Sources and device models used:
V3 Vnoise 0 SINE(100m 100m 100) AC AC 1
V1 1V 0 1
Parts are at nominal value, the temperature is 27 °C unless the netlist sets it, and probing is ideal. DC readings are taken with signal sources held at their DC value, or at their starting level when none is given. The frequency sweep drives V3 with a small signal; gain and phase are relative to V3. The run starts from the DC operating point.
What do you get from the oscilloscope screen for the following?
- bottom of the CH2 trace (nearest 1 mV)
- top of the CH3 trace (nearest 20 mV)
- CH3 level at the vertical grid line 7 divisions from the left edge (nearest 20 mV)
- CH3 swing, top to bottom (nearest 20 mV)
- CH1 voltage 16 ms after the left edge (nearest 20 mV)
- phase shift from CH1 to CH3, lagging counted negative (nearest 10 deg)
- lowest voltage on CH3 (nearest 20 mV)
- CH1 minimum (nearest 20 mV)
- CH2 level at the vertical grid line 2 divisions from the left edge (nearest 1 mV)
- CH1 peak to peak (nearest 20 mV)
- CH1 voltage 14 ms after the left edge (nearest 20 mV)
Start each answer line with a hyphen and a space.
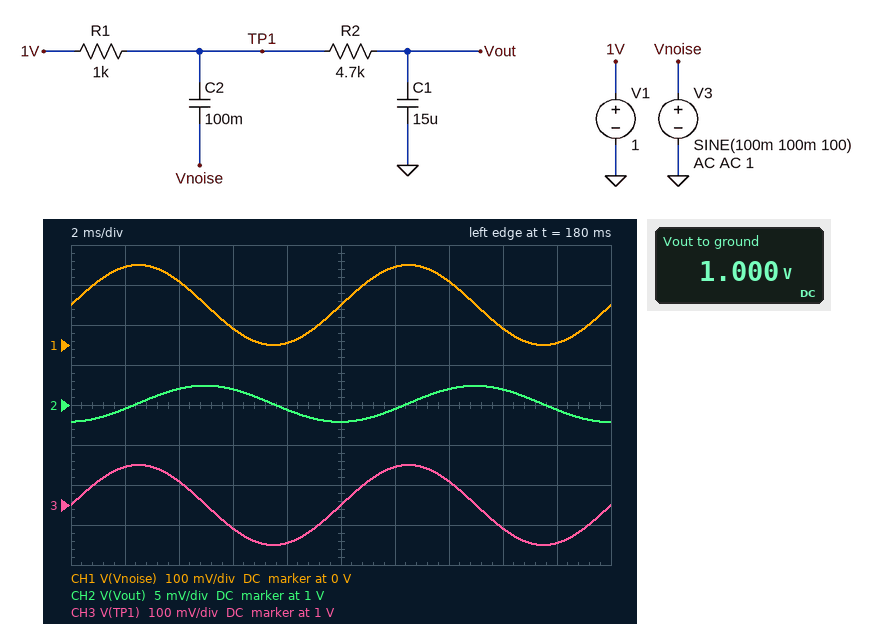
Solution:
- 998 mV
- 1.10 V
- 1.06 V
- 200 mV
- 40 mV
- 0 deg
- 900 mV
- 0 V
- 1.002 V
- 200 mV
- 160 mV
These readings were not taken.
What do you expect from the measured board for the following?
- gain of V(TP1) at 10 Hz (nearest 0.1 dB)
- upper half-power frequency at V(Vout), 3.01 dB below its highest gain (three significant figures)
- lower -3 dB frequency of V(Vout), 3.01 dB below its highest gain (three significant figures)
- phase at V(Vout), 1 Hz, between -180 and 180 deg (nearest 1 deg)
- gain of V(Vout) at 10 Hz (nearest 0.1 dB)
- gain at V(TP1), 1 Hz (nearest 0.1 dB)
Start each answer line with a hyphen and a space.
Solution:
- 0 dB
- 2.26 Hz
- 1.59 mHz
- -24 deg
- -13.1 dB
- 0 dB
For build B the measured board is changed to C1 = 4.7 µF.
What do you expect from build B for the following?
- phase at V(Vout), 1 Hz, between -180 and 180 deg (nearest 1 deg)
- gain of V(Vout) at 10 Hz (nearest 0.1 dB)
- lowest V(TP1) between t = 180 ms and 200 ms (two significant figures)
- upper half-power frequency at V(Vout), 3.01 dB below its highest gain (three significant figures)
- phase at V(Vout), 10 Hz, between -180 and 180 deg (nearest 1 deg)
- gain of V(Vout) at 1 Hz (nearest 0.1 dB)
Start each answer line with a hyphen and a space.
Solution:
- -8 deg
- -4.7 dB
- 900 mV
- 7.21 Hz
- -54 deg
- -0.1 dB
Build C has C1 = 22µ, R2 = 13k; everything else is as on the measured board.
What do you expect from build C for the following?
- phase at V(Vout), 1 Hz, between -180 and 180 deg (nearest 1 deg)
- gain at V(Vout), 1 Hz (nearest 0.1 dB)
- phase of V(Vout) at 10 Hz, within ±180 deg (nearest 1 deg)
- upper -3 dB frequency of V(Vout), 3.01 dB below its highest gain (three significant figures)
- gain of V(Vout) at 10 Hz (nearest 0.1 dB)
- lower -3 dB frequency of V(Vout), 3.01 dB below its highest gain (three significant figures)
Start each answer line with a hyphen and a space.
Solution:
- -61 deg
- -6.3 dB
- -87 deg
- 560 mHz
- -25.1 dB
- 1.58 mHz
